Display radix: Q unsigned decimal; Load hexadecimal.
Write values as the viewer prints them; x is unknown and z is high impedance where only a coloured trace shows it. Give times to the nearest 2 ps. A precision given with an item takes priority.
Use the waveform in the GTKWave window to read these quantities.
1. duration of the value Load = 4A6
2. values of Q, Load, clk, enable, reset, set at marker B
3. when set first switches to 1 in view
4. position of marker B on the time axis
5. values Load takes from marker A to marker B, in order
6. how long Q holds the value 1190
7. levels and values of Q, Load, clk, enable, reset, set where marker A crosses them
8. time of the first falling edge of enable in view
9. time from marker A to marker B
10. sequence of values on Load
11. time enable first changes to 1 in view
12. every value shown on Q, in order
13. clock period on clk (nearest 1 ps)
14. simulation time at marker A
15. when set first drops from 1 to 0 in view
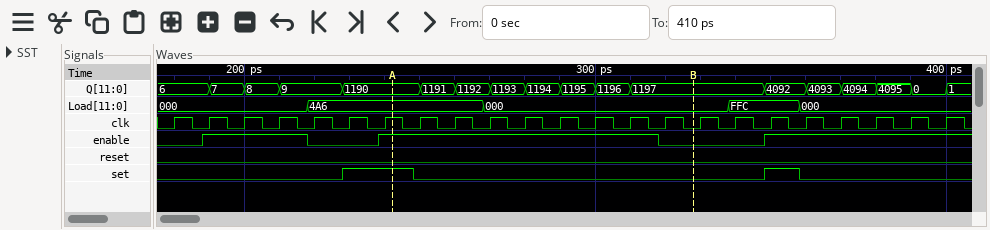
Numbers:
50 ps
Q=1197, Load=000, clk=0, enable=0, reset=0, set=0
228 ps
328 ps
4A6, 000
22 ps
Q=1190, Load=4A6, clk=1, enable=1, reset=0, set=1
218 ps
86 ps
000, 4A6, 000, FFC, 000
188 ps
6, 7, 8, 9, 1190, 1191, 1192, 1193, 1194, 1195, 1196, 1197, 4092, 4093, 4094, 4095, 0, 1
10 ps
242 ps
248 ps
